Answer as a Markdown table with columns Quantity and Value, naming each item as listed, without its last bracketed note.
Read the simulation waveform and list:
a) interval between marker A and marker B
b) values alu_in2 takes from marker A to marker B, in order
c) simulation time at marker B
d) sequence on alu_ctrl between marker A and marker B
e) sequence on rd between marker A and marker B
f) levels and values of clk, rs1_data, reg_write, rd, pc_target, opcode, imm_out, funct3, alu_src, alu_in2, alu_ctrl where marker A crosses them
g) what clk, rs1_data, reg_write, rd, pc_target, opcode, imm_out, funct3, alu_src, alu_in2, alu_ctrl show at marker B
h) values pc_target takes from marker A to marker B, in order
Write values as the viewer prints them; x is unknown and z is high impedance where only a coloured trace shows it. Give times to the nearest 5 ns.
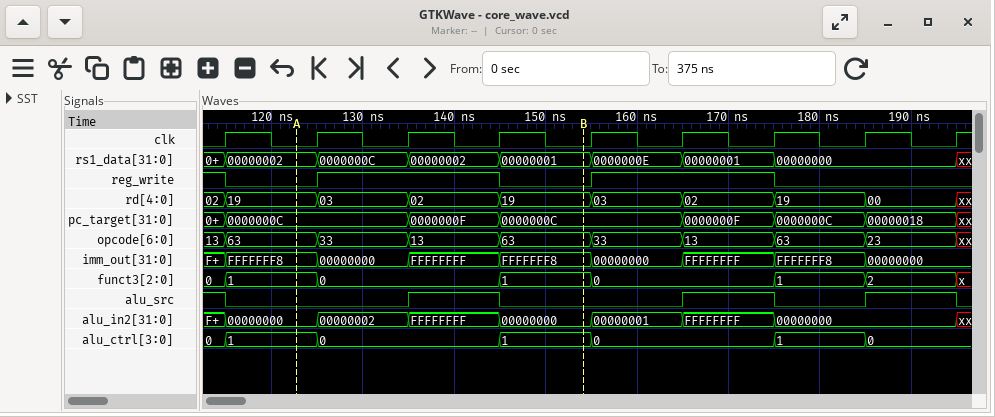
| Quantity | Value |
|---|---|
| interval between marker A and marker B | 30 ns |
| values alu_in2 takes from marker A to marker B, in order | 00000000, 00000002, FFFFFFFF, 00000000 |
| simulation time at marker B | 155 ns |
| sequence on alu_ctrl between marker A and marker B | 1, 0, 1 |
| sequence on rd between marker A and marker B | 19, 03, 02, 19 |
| levels and values of clk, rs1_data, reg_write, rd, pc_target, opcode, imm_out, funct3, alu_src, alu_in2, alu_ctrl where marker A crosses them | clk=0, rs1_data=00000002, reg_write=0, rd=19, pc_target=0000000C, opcode=63, imm_out=FFFFFFF8, funct3=1, alu_src=0, alu_in2=00000000, alu_ctrl=1 |
| what clk, rs1_data, reg_write, rd, pc_target, opcode, imm_out, funct3, alu_src, alu_in2, alu_ctrl show at marker B | clk=0, rs1_data=00000001, reg_write=0, rd=19, pc_target=0000000C, opcode=63, imm_out=FFFFFFF8, funct3=1, alu_src=0, alu_in2=00000000, alu_ctrl=1 |
| values pc_target takes from marker A to marker B, in order | 0000000C, 0000000F, 0000000C |
